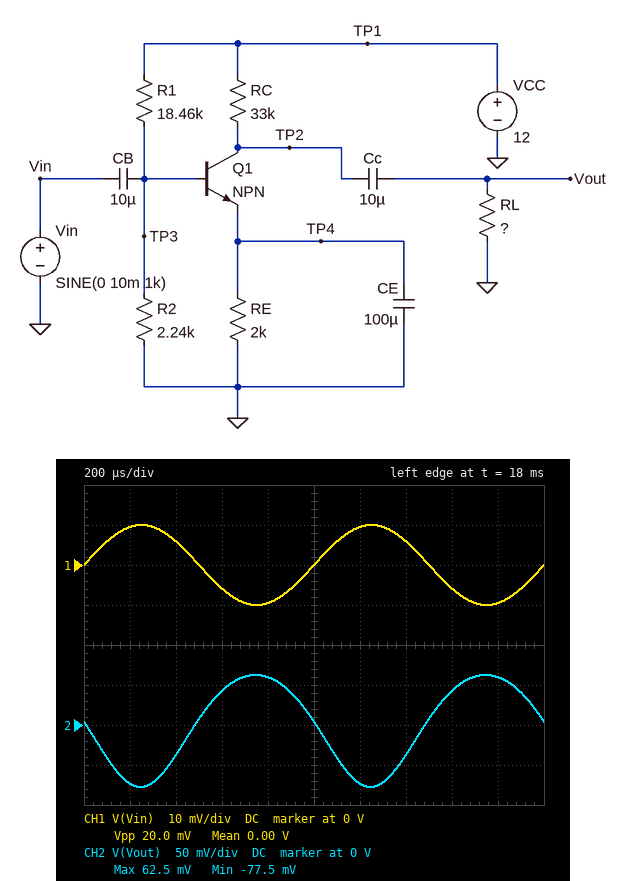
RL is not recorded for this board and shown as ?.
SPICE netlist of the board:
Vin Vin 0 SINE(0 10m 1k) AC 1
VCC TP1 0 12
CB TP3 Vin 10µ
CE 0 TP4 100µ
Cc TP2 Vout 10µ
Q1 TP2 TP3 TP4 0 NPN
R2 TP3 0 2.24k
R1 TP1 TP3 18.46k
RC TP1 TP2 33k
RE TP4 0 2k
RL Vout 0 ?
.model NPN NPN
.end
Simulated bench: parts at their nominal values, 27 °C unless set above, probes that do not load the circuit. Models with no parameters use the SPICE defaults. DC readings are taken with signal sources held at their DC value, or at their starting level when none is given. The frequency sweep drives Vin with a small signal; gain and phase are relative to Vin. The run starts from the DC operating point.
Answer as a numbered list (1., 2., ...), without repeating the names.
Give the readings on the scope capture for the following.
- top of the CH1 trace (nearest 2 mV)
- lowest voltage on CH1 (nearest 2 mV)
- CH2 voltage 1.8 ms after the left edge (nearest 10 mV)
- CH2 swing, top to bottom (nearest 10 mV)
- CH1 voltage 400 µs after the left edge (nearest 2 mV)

1. 10 mV
2. -10 mV
3. 60 mV
4. 140 mV
5. 6 mV
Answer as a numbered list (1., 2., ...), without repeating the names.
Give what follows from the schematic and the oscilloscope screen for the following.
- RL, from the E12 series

1. 680 Ω
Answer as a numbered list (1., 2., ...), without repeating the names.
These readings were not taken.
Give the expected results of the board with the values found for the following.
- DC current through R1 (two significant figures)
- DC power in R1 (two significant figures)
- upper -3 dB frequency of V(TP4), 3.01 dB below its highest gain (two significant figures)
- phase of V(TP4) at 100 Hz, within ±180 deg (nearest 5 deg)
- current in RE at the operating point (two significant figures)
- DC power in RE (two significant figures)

1. 580 µA
2. 6.2 mW
3. 32 Hz
4. -75 deg
5. 280 µA
6. 150 µW
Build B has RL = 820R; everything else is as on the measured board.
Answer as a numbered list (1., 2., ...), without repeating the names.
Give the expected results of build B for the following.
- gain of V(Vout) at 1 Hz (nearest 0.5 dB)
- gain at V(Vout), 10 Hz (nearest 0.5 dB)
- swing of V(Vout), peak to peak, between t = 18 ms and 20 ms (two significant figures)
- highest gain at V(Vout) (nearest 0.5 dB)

1. -23.5 dB
2. 9.5 dB
3. 170 mV
4. 18.5 dB
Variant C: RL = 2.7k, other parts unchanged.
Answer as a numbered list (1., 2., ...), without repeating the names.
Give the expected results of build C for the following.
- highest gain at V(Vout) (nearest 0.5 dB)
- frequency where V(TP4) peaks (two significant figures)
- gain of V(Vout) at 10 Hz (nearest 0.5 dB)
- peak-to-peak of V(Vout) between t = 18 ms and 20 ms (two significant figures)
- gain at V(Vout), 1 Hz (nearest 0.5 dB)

1. 28.5 dB
2. 12 Hz
3. 19.5 dB
4. 520 mV
5. -13.5 dB
